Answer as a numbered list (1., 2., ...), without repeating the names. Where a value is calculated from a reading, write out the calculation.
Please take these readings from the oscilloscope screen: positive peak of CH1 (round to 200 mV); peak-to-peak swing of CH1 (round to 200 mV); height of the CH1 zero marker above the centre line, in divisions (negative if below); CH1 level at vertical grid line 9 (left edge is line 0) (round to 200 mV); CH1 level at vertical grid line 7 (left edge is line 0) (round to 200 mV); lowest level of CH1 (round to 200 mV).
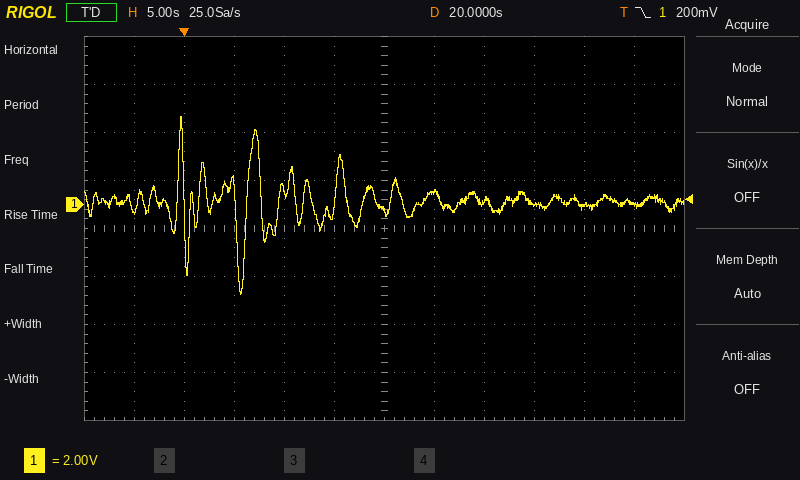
1. 3.6 V
2. 3.6 V − (-3.8 V) = 7.4 V
3. +0.5 div
4. 0.0 V
5. 600 mV
6. -3.8 V
